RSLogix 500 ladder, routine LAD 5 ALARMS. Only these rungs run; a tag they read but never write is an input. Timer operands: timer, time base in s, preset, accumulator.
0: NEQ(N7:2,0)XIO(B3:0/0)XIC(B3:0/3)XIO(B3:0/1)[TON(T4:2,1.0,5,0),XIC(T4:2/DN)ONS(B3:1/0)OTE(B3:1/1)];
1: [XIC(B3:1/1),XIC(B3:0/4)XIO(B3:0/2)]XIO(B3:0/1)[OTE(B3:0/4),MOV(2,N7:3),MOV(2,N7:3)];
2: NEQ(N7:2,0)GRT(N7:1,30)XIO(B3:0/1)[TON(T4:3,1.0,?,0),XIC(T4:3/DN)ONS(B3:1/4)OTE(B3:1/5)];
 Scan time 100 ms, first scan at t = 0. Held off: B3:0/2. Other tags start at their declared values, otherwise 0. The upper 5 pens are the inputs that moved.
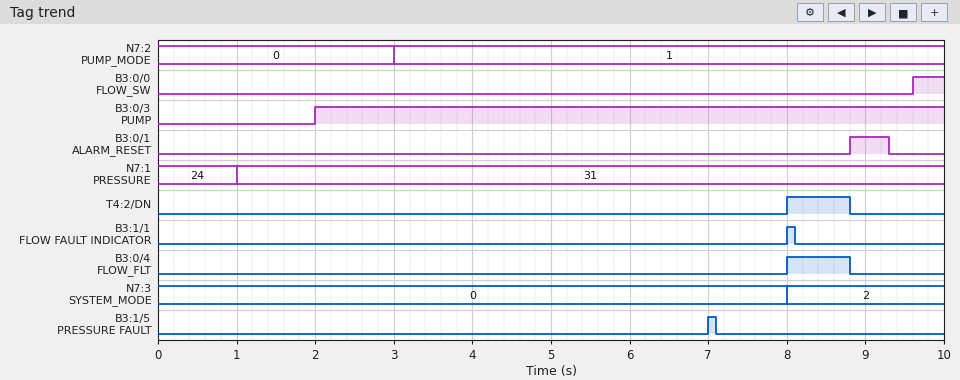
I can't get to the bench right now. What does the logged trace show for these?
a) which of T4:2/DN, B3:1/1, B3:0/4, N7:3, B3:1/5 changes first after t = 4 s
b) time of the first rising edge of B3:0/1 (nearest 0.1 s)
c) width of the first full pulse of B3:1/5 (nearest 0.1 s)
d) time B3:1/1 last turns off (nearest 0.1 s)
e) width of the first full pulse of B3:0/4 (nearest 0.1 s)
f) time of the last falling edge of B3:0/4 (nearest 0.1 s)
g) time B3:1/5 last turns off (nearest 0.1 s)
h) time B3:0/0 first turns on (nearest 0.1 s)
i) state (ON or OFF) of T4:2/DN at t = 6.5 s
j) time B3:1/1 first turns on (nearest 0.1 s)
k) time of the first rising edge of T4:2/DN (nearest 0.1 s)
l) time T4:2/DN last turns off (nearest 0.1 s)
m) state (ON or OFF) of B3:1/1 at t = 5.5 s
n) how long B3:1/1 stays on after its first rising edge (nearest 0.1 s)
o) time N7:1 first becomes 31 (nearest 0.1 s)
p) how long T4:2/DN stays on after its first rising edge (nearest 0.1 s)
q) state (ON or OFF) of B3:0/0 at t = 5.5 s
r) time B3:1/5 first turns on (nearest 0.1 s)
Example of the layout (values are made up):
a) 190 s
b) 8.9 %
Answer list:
a) B3:1/5
b) 8.8 s
c) 0.1 s
d) 8.1 s
e) 0.8 s
f) 8.8 s
g) 7.1 s
h) 9.6 s
i) OFF
j) 8.0 s
k) 8.0 s
l) 8.8 s
m) OFF
n) 0.1 s
o) 1.0 s
p) 0.8 s
q) OFF
r) 7.0 s
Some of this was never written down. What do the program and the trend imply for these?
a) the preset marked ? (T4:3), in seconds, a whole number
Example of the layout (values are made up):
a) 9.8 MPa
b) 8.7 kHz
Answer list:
a) 4 s
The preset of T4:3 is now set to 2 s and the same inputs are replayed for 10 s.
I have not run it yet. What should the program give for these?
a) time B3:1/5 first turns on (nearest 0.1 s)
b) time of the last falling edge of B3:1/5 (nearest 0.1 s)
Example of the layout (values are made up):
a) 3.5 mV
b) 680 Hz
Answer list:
a) 5.0 s
b) 5.1 s
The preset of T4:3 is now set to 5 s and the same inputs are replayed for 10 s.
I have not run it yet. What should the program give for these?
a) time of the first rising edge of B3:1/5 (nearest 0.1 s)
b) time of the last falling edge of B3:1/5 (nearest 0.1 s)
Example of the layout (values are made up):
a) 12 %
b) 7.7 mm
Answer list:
a) 8.0 s
b) 8.1 s
